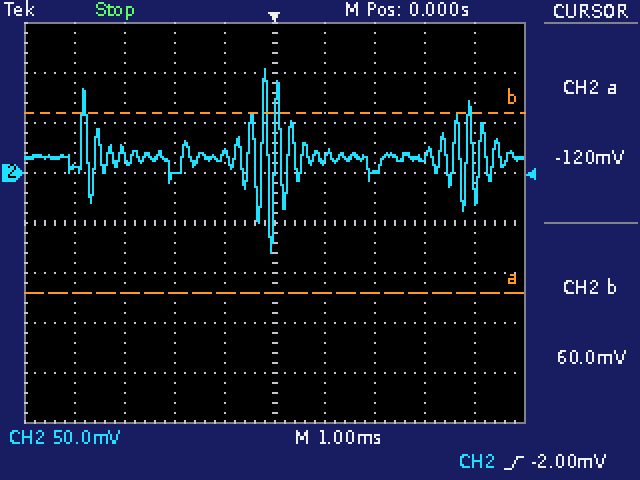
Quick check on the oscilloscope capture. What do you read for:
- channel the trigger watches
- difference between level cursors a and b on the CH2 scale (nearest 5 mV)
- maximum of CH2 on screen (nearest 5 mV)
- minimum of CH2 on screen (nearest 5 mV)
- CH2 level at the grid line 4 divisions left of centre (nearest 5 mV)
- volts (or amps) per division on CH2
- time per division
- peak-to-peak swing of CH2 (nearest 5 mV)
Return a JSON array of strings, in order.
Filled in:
["CH2", "180 mV", "105 mV", "-80 mV", "5 mV", "50 mV", "1 ms", "185 mV"]
